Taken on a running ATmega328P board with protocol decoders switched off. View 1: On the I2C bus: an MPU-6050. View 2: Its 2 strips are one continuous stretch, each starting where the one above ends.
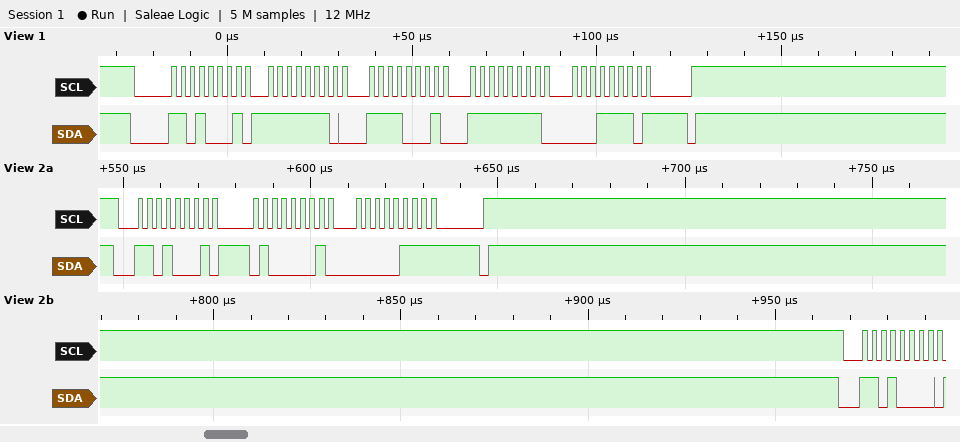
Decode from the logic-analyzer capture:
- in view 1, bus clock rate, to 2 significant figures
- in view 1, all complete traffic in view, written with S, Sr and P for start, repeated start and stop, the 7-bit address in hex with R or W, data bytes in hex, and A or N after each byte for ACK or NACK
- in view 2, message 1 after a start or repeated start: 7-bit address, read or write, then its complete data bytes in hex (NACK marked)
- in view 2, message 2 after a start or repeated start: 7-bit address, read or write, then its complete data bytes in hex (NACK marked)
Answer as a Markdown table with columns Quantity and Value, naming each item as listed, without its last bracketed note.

| Quantity | Value |
|---|---|
| in view 1, bus clock rate, to 2 significant figures | 400 kHz |
| in view 1, all complete traffic in view, written with S, Sr and P for start, repeated start and stop, the 7-bit address in hex with R or W, data bytes in hex, and A or N after each byte for ACK or NACK | S 68R A FE A F1 A FF A 1E N P |
| in view 2, message 1 after a start or repeated start: 7-bit address, read or write, then its complete data bytes in hex | 0x68 read: 41 07 NACK |
| in view 2, message 2 after a start or repeated start: 7-bit address, read or write, then its complete data bytes in hex | 0x68 write |
